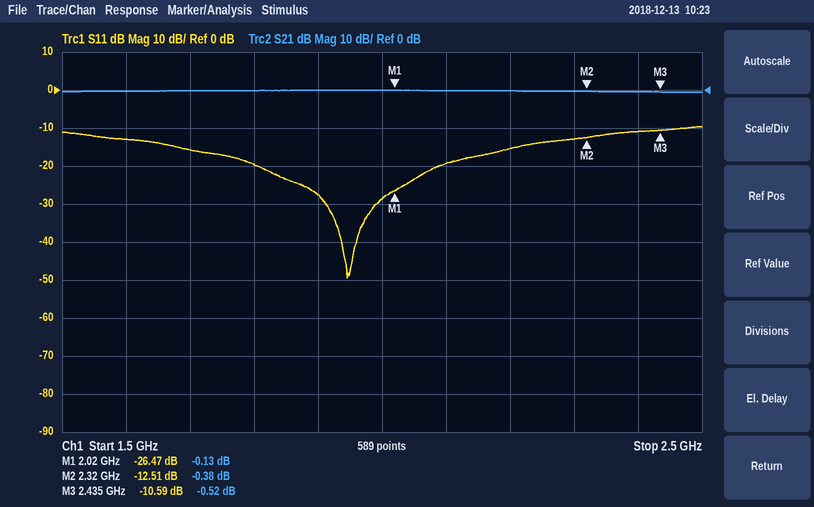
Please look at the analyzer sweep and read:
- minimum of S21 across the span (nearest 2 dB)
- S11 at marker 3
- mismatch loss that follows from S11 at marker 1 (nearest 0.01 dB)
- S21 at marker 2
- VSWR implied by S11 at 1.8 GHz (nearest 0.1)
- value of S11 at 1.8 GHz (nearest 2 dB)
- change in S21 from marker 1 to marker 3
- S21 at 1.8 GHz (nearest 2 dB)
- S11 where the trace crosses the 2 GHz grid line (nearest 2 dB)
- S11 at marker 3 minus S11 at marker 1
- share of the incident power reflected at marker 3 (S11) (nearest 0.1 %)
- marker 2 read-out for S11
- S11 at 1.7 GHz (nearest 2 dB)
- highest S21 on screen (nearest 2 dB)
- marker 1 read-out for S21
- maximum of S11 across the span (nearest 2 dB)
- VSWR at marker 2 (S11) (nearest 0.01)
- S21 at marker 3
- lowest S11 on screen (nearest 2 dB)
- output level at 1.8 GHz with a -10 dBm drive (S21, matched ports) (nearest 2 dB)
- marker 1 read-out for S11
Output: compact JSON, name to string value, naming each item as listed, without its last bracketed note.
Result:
{"minimum of S21 across the span": "0 dB", "S11 at marker 3": "-10.59 dB", "mismatch loss that follows from S11 at marker 1": "0.01 dB", "S21 at marker 2": "-0.38 dB", "VSWR implied by S11 at 1.8 GHz": "1.2", "value of S11 at 1.8 GHz": "-20 dB", "change in S21 from marker 1 to marker 3": "-0.39 dB", "S21 at 1.8 GHz": "0 dB", "S11 where the trace crosses the 2 GHz grid line": "-28 dB", "S11 at marker 3 minus S11 at marker 1": "15.88 dB", "share of the incident power reflected at marker 3 (S11)": "8.7 %", "marker 2 read-out for S11": "-12.51 dB", "S11 at 1.7 GHz": "-16 dB", "highest S21 on screen": "0 dB", "marker 1 read-out for S21": "-0.13 dB", "maximum of S11 across the span": "-10 dB", "VSWR at marker 2 (S11)": "1.62", "S21 at marker 3": "-0.52 dB", "lowest S11 on screen": "-50 dB", "output level at 1.8 GHz with a -10 dBm drive (S21, matched ports)": "-10 dBm", "marker 1 read-out for S11": "-26.47 dB"}
